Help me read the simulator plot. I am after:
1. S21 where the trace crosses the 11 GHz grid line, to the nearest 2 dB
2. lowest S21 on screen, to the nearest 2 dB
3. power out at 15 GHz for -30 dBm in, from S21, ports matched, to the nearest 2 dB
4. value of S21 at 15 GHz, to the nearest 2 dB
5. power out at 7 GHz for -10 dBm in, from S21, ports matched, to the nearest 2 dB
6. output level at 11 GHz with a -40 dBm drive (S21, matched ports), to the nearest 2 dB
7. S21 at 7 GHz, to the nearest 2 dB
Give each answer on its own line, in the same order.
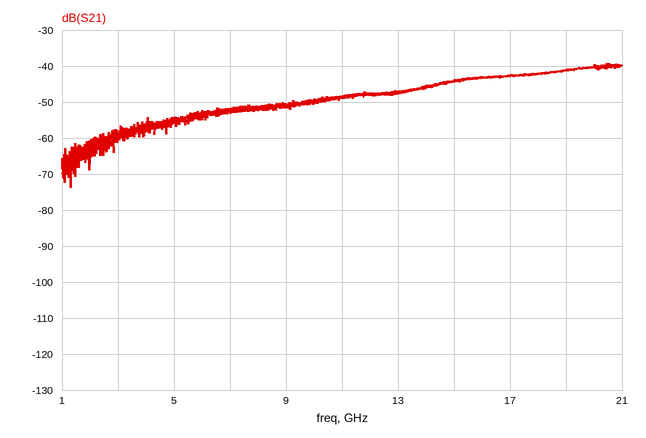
-48 dB
-74 dB
-74 dBm
-44 dB
-62 dBm
-88 dBm
-52 dB
